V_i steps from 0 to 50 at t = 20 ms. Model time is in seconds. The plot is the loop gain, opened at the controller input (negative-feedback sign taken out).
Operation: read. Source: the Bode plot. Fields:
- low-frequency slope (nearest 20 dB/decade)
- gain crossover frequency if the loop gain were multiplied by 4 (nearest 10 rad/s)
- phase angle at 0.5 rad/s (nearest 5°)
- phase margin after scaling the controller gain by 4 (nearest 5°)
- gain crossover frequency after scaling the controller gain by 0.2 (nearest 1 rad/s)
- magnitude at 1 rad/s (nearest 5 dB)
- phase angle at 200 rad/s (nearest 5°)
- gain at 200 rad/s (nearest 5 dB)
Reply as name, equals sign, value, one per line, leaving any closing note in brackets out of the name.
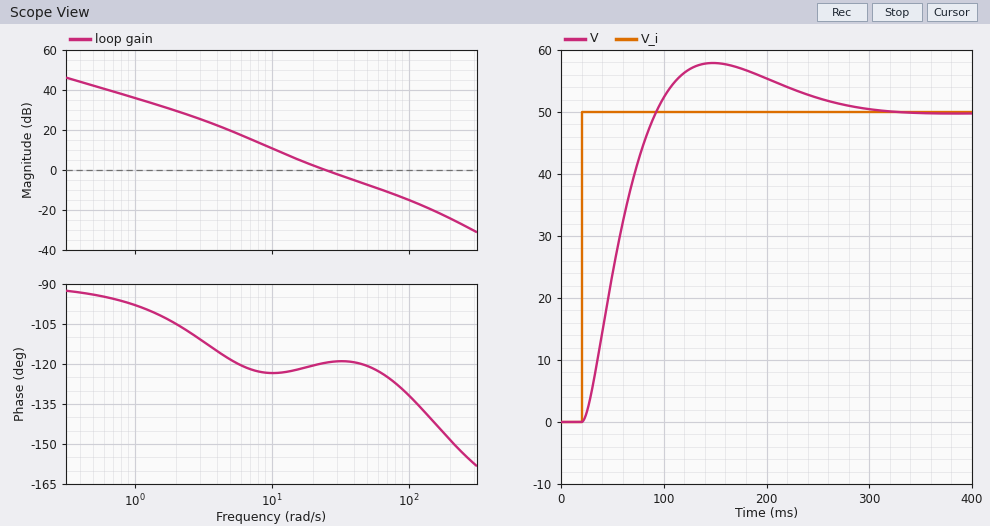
low-frequency slope = -20 dB/decade
gain crossover frequency if the loop gain were multiplied by 4 = 80 rad/s
phase angle at 0.5 rad/s = -95°
phase margin after scaling the controller gain by 4 = 55°
gain crossover frequency after scaling the controller gain by 0.2 = 8 rad/s
magnitude at 1 rad/s = 35 dB
phase angle at 200 rad/s = -150°
gain at 200 rad/s = -25 dB
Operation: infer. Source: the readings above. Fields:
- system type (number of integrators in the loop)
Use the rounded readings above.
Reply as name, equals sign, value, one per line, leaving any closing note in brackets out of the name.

system type = 1
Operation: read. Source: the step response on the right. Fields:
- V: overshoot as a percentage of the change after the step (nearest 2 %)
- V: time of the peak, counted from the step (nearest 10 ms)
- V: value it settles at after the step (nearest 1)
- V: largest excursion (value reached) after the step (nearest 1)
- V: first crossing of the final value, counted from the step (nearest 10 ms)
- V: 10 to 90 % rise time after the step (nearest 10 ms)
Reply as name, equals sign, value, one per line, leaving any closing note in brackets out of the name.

V: overshoot as a percentage of the change after the step = 16 %
V: time of the peak, counted from the step = 130 ms
V: value it settles at after the step = 50
V: largest excursion (value reached) after the step = 58
V: first crossing of the final value, counted from the step = 70 ms
V: 10 to 90 % rise time after the step = 50 ms
